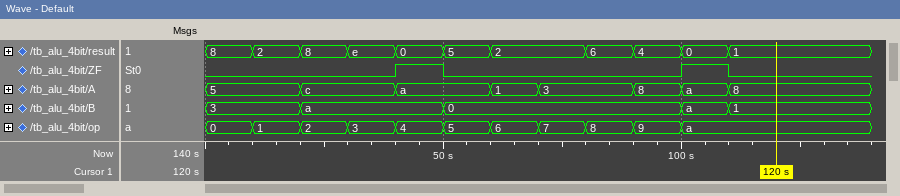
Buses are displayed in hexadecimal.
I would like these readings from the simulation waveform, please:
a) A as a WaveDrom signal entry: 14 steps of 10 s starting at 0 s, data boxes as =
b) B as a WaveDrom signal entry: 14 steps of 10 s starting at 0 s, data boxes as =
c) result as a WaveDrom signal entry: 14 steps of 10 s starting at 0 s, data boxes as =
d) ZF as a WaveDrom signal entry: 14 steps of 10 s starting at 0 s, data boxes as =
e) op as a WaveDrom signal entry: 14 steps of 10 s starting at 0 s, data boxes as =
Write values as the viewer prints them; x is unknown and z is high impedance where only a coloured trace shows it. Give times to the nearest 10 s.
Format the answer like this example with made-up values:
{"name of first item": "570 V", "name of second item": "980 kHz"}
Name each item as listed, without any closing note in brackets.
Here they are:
{"A as a WaveDrom signal entry: 14 steps of 10 s starting at 0 s, data boxes as =": "{name: 'A', wave: '=.=.=.==.===..', data: '5 c a 1 3 8 a 8'}", "B as a WaveDrom signal entry: 14 steps of 10 s starting at 0 s, data boxes as =": "{name: 'B', wave: '=.=..=....==..', data: '3 a 0 a 1'}", "result as a WaveDrom signal entry: 14 steps of 10 s starting at 0 s, data boxes as =": "{name: 'result', wave: '=======.====..', data: '8 2 8 e 0 5 2 6 4 0 1'}", "ZF as a WaveDrom signal entry: 14 steps of 10 s starting at 0 s, data boxes as =": "{name: 'ZF', wave: '0...10....10..'}", "op as a WaveDrom signal entry: 14 steps of 10 s starting at 0 s, data boxes as =": "{name: 'op', wave: '===========...', data: '0 1 2 3 4 5 6 7 8 9 a'}"}
